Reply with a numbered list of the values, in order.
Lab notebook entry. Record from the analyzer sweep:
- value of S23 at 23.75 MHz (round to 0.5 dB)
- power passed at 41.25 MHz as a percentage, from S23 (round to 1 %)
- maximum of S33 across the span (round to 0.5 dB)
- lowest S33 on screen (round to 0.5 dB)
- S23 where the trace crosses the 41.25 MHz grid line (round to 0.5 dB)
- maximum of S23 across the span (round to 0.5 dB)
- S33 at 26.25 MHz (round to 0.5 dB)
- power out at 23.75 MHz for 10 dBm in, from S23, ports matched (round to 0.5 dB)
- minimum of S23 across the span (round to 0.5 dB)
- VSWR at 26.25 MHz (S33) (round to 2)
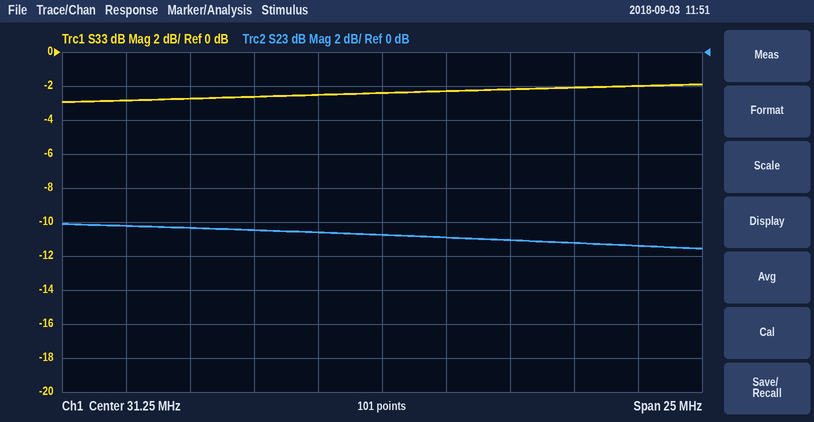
1. -10.5 dB
2. 7 %
3. -2.0 dB
4. -3.0 dB
5. -11.5 dB
6. -10.0 dB
7. -2.5 dB
8. -0.5 dBm
9. -11.5 dB
10. 6
